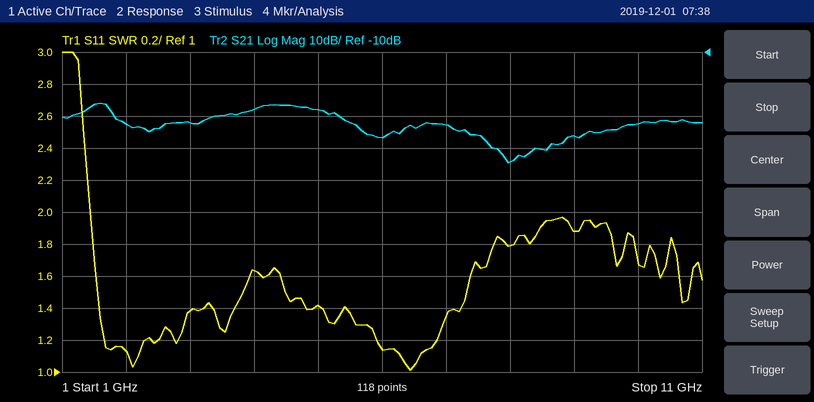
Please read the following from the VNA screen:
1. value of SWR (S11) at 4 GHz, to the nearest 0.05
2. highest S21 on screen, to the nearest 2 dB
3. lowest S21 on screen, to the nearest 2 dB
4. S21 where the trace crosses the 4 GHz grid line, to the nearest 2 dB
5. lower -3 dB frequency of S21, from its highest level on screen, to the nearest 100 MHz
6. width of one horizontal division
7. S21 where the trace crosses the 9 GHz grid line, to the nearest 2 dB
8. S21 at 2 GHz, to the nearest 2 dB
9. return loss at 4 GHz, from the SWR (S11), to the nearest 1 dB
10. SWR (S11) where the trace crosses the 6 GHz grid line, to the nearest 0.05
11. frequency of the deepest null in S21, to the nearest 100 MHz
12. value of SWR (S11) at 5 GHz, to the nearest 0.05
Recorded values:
1.65
-26 dB
-44 dB
-28 dB
1.3 GHz
1 GHz
-36 dB
-32 dB
12 dB
1.15
8.0 GHz
1.40
